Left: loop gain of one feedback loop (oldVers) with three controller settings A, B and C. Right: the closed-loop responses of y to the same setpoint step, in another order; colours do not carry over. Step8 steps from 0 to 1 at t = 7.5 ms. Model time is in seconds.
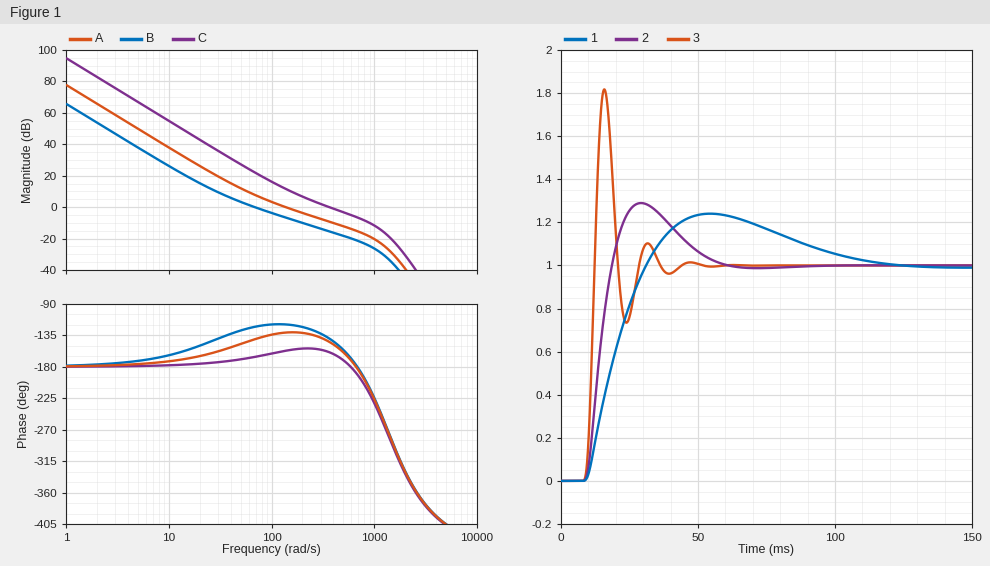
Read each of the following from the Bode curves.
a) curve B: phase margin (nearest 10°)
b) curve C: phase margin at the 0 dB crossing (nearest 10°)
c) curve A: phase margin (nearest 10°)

60°
20°
50°
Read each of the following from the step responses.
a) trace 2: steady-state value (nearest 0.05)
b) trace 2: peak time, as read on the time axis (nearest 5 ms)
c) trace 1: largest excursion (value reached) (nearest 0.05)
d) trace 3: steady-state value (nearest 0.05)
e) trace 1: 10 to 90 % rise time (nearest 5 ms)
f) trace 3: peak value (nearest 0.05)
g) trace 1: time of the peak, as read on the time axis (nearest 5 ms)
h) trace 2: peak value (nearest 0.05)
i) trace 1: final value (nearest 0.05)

1.00
30 ms
1.25
1.00
15 ms
1.80
55 ms
1.30
1.00
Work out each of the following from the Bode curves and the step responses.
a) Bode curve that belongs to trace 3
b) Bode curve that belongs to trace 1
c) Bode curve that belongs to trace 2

C
B
A
